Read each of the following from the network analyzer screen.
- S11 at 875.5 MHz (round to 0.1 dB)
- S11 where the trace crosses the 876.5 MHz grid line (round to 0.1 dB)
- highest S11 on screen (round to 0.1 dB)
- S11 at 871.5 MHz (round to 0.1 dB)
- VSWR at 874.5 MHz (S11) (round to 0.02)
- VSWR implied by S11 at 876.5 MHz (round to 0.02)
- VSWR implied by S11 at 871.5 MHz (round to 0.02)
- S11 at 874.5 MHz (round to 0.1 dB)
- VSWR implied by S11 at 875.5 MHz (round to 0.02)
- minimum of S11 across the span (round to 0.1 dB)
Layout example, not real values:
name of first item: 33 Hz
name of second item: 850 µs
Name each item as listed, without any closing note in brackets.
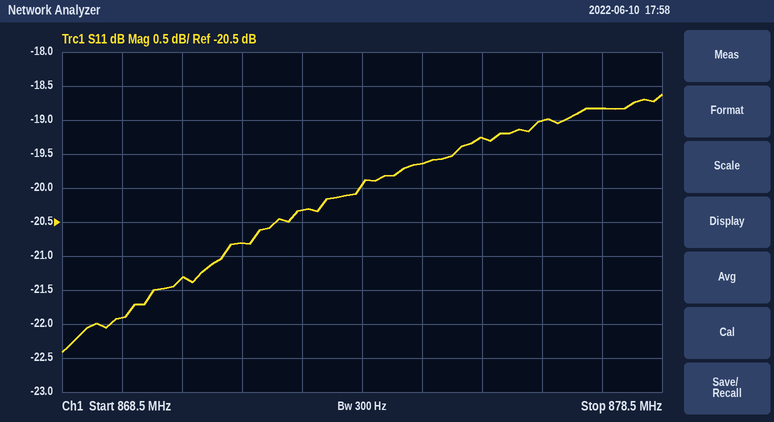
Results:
S11 at 875.5 MHz: -19.3 dB
S11 where the trace crosses the 876.5 MHz grid line: -19.0 dB
highest S11 on screen: -18.6 dB
S11 at 871.5 MHz: -20.8 dB
VSWR at 874.5 MHz (S11): 1.24
VSWR implied by S11 at 876.5 MHz: 1.26
VSWR implied by S11 at 871.5 MHz: 1.20
S11 at 874.5 MHz: -19.6 dB
VSWR implied by S11 at 875.5 MHz: 1.24
minimum of S11 across the span: -22.4 dB
